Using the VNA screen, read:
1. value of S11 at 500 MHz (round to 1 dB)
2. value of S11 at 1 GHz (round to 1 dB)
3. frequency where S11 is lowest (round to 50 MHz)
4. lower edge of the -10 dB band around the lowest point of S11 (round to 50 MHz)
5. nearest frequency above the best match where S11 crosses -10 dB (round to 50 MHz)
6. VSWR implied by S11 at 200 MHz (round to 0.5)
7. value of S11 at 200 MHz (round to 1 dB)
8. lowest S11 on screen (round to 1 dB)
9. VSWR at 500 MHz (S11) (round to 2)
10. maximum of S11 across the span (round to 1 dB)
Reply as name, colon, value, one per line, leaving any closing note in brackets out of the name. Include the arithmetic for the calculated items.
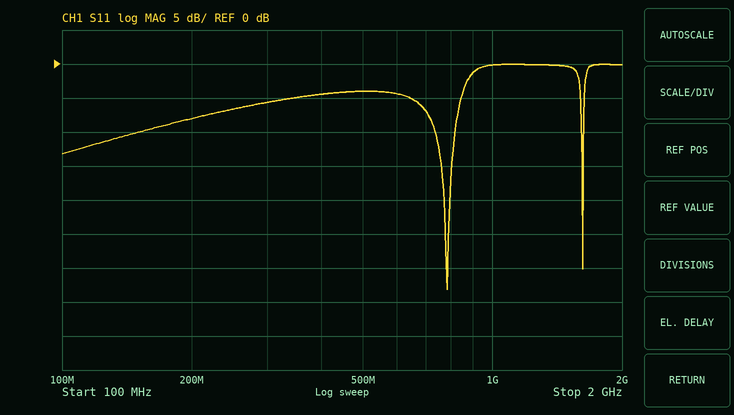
value of S11 at 500 MHz: -4 dB
value of S11 at 1 GHz: 0 dB
frequency where S11 is lowest: 800 MHz
lower edge of the -10 dB band around the lowest point of S11: 750 MHz
nearest frequency above the best match where S11 crosses -10 dB: 800 MHz
VSWR implied by S11 at 200 MHz: |Γ| = 10^(-8/20) = 0.3981; VSWR = (1 + 0.3981)/(1 − 0.3981) ≈ 2.32, so 2.5 to the nearest 0.5
value of S11 at 200 MHz: -8 dB
lowest S11 on screen: -33 dB
VSWR at 500 MHz (S11): |Γ| = 10^(-4/20) = 0.6310; VSWR = (1 + 0.6310)/(1 − 0.6310) ≈ 4
maximum of S11 across the span: 0 dB
